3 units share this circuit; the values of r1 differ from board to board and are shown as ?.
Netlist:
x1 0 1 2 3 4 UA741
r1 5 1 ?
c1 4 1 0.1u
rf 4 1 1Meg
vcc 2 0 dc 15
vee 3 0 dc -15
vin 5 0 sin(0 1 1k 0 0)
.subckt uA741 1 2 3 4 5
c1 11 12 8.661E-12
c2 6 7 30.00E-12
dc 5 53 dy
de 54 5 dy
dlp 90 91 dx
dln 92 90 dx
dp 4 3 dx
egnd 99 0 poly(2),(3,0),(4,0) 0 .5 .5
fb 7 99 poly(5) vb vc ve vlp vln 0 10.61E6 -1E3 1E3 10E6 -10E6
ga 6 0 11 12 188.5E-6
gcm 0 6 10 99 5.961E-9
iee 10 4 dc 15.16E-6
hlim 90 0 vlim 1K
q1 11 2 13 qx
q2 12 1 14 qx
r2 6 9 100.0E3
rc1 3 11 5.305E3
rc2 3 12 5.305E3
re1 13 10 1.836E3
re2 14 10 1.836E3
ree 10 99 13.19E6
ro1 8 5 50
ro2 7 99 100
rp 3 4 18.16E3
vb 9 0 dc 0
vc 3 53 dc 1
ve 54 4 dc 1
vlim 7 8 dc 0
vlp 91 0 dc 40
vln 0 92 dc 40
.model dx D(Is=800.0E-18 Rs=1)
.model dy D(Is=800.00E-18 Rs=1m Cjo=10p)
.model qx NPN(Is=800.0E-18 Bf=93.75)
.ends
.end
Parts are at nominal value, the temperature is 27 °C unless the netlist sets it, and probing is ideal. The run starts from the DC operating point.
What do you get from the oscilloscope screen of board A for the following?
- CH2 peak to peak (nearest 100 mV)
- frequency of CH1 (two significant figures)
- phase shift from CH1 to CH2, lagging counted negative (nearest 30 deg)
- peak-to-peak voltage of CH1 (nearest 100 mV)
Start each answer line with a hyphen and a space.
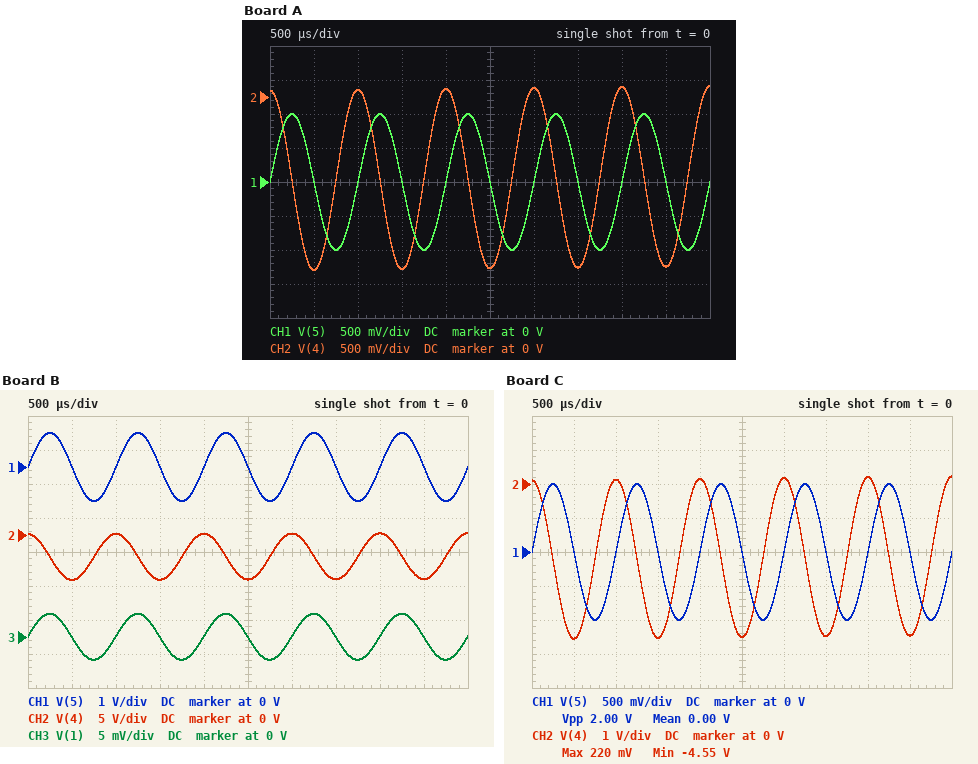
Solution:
- 2.7 V
- 1.0 kHz
- 90 deg
- 2.0 V
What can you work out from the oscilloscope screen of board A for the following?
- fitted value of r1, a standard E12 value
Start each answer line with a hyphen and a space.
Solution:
- 1.2 kΩ
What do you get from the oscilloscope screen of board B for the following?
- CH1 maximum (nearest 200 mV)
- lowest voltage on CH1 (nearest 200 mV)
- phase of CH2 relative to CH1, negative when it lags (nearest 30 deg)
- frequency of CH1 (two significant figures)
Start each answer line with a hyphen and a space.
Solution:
- 1.0 V
- -1.0 V
- 90 deg
- 1.0 kHz
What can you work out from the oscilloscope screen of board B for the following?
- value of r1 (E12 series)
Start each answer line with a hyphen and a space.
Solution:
- 470 Ω
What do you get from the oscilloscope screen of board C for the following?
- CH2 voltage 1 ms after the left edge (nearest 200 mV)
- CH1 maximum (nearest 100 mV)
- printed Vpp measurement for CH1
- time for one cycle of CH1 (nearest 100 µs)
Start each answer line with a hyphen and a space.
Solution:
- 200 mV
- 1.0 V
- 2.00 V
- 1.0 ms
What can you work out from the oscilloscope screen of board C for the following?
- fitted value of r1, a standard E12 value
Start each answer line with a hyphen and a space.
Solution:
- 680 Ω
